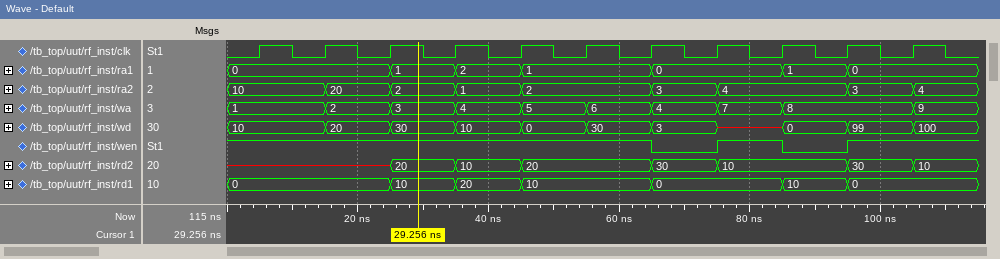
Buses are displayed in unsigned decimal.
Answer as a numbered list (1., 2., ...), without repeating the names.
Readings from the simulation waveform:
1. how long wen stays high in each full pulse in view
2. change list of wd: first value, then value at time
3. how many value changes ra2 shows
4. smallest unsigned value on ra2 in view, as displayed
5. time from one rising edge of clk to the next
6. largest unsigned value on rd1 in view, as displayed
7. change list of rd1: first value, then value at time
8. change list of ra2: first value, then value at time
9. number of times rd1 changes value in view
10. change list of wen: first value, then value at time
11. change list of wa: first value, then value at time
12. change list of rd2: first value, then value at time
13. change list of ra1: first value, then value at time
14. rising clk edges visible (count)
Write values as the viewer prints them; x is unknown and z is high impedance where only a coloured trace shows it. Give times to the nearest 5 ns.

1. 10 ns
2. 10, 20 at 15 ns, 30 at 25 ns, 10 at 35 ns, 0 at 45 ns, 30 at 55 ns, 3 at 65 ns, x at 75 ns, 0 at 85 ns, 99 at 95 ns, 100 at 105 ns
3. 8
4. 1
5. 10 ns
6. 20
7. 0, 10 at 25 ns, 20 at 35 ns, 10 at 45 ns, 0 at 65 ns, 10 at 85 ns, 0 at 95 ns
8. 10, 20 at 15 ns, 2 at 25 ns, 1 at 35 ns, 2 at 45 ns, 3 at 65 ns, 4 at 75 ns, 3 at 95 ns, 4 at 105 ns
9. 6
10. 1, 0 at 65 ns, 1 at 75 ns, 0 at 85 ns, 1 at 95 ns
11. 1, 2 at 15 ns, 3 at 25 ns, 4 at 35 ns, 5 at 45 ns, 6 at 55 ns, 4 at 65 ns, 7 at 75 ns, 8 at 85 ns, 9 at 105 ns
12. x, 20 at 25 ns, 10 at 35 ns, 20 at 45 ns, 30 at 65 ns, 10 at 75 ns, 30 at 95 ns, 10 at 105 ns
13. 0, 1 at 25 ns, 2 at 35 ns, 1 at 45 ns, 0 at 65 ns, 1 at 85 ns, 0 at 95 ns
14. 11
